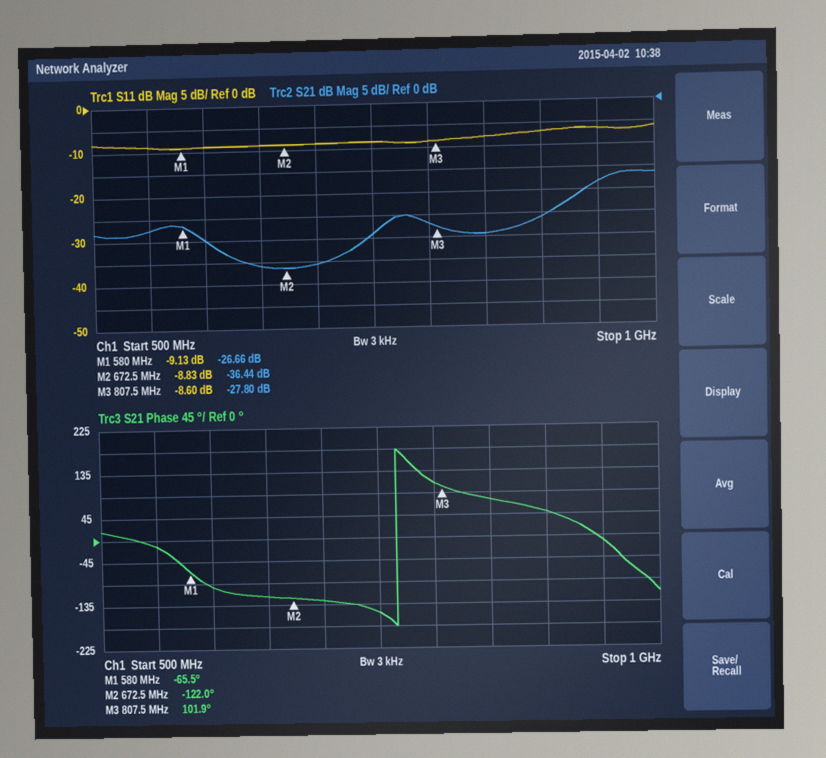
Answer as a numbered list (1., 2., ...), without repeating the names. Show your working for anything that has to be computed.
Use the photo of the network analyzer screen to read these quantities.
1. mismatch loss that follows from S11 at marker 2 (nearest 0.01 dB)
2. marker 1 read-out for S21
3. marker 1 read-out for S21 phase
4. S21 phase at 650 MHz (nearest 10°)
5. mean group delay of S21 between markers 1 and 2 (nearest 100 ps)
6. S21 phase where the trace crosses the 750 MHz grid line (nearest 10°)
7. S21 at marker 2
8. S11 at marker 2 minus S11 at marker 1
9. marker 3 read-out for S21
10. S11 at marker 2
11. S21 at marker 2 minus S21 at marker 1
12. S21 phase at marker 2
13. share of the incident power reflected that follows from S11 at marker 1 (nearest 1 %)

1. −10 log10(1 − 10^(-8.83/10)) ≈ 0.61 dB
2. -26.66 dB
3. -65.5°
4. -120°
5. −(-122° − (-65.5°))/(360° × 92.5 MHz) ≈ 1.7 ns
6. -150°
7. -36.44 dB
8. -8.83 − (-9.13) = 0.30 dB
9. -27.80 dB
10. -8.83 dB
11. -36.44 − (-26.66) = -9.78 dB
12. -122.0°
13. 10^(-9.13/10) ≈ 12 %
